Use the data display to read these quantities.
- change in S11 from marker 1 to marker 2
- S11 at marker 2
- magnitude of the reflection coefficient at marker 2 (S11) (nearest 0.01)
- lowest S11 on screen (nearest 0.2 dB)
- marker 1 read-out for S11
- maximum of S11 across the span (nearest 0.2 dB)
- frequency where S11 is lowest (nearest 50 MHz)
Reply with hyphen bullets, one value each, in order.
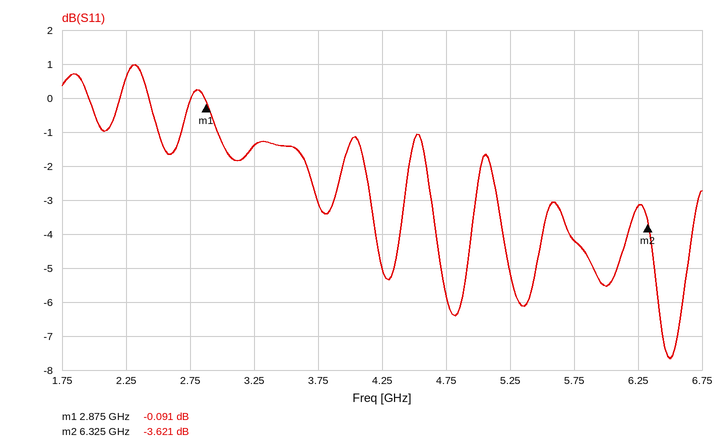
- -3.530 dB
- -3.621 dB
- 0.66
- -7.6 dB
- -0.091 dB
- 1.0 dB
- 6.50 GHz
